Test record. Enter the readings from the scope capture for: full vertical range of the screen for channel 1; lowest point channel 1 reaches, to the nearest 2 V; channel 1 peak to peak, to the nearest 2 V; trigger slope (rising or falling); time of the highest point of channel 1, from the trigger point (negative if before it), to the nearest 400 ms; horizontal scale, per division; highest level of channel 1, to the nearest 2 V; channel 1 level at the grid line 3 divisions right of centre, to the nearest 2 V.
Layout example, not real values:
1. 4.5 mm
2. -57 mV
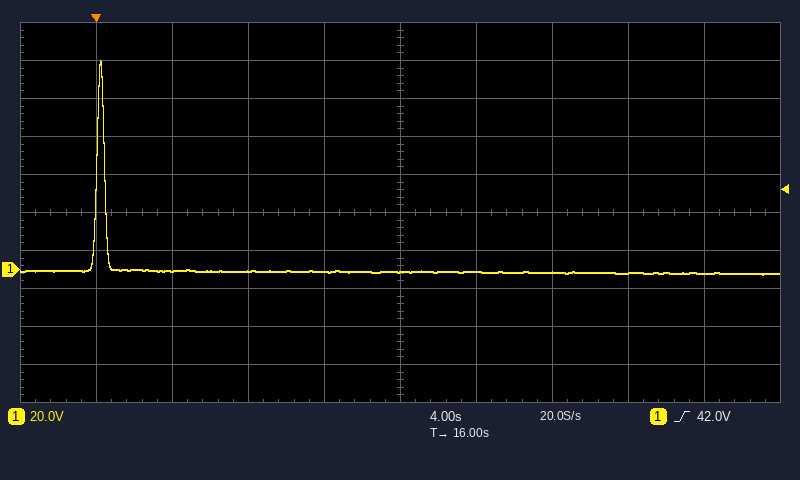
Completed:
1. 200 V
2. -2 V
3. 112 V
4. rising
5. +400 ms
6. 4 s
7. 110 V
8. -2 V
